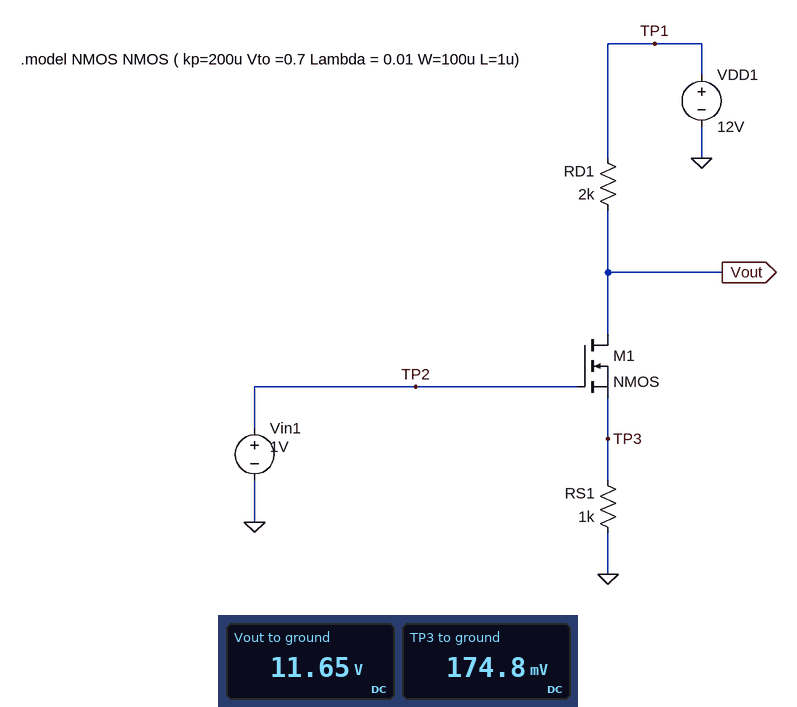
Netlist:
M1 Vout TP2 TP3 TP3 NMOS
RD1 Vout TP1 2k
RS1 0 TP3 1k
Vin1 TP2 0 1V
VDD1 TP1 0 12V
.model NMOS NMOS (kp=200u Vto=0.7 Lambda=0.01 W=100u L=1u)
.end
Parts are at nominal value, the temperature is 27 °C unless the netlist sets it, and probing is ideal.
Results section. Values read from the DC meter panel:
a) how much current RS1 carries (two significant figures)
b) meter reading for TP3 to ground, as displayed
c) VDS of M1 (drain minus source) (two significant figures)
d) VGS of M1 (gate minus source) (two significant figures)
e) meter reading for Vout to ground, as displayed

170 µA
174.8 mV
11 V
830 mV
11.65 V
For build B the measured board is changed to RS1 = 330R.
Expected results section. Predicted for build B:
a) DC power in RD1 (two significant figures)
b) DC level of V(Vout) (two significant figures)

260 µW
11 V
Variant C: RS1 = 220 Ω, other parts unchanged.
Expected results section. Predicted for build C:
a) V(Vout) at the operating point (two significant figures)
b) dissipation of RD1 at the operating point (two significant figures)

11 V
400 µW
